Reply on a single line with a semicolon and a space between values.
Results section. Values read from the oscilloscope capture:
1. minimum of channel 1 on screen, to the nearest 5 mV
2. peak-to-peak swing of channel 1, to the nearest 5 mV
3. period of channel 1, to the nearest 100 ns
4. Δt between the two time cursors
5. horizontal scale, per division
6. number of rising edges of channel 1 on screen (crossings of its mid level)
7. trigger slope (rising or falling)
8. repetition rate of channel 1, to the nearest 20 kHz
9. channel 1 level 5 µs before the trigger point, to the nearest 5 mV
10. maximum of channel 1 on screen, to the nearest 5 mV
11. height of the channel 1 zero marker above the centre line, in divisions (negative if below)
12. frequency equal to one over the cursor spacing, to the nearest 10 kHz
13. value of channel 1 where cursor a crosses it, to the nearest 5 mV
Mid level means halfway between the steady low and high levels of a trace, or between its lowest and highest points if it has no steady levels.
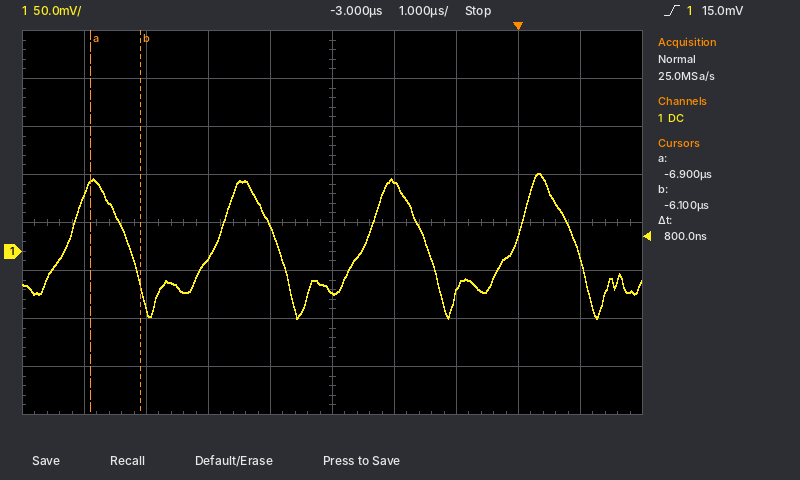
-70 mV; 150 mV; 2.4 µs; 800 ns; 1 µs; 4; rising; 420 kHz; -5 mV; 80 mV; -0.6 div; 1.25 MHz; 70 mV
